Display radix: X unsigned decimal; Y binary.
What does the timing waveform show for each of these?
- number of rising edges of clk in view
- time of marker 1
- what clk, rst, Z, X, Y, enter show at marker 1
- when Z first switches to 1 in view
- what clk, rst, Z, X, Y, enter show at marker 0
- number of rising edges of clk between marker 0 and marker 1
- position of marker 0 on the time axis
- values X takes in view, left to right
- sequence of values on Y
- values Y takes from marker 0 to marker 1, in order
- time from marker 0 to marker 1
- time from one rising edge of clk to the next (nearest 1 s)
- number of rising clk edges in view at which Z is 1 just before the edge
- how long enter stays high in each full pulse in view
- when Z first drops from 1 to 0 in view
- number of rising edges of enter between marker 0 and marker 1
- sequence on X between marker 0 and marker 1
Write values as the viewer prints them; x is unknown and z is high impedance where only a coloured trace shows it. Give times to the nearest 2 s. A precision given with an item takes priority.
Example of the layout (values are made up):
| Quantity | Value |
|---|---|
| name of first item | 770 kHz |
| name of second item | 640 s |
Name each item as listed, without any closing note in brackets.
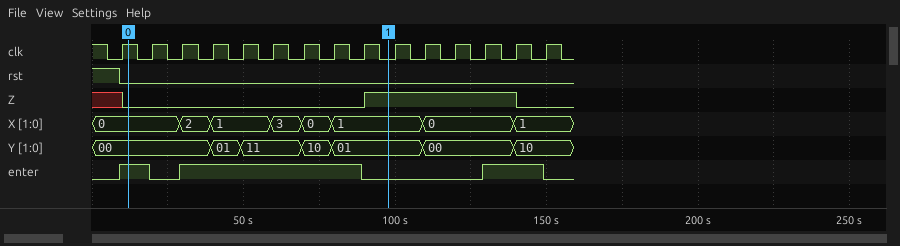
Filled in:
| Quantity | Value |
|---|---|
| number of rising edges of clk in view | 15 |
| time of marker 1 | 98 s |
| what clk, rst, Z, X, Y, enter show at marker 1 | clk=0, rst=0, Z=1, X=1, Y=01, enter=0 |
| when Z first switches to 1 in view | 90 s |
| what clk, rst, Z, X, Y, enter show at marker 0 | clk=1, rst=0, Z=0, X=0, Y=00, enter=1 |
| number of rising edges of clk between marker 0 and marker 1 | 8 |
| position of marker 0 on the time axis | 12 s |
| values X takes in view, left to right | 0, 2, 1, 3, 0, 1, 0, 1 |
| sequence of values on Y | 00, 01, 11, 10, 01, 00, 10 |
| values Y takes from marker 0 to marker 1, in order | 00, 01, 11, 10, 01 |
| time from marker 0 to marker 1 | 86 s |
| time from one rising edge of clk to the next | 10 s |
| number of rising clk edges in view at which Z is 1 just before the edge | 5 |
| how long enter stays high in each full pulse in view | 10 s, 60 s, 20 s |
| when Z first drops from 1 to 0 in view | 140 s |
| number of rising edges of enter between marker 0 and marker 1 | 1 |
| sequence on X between marker 0 and marker 1 | 0, 2, 1, 3, 0, 1 |
